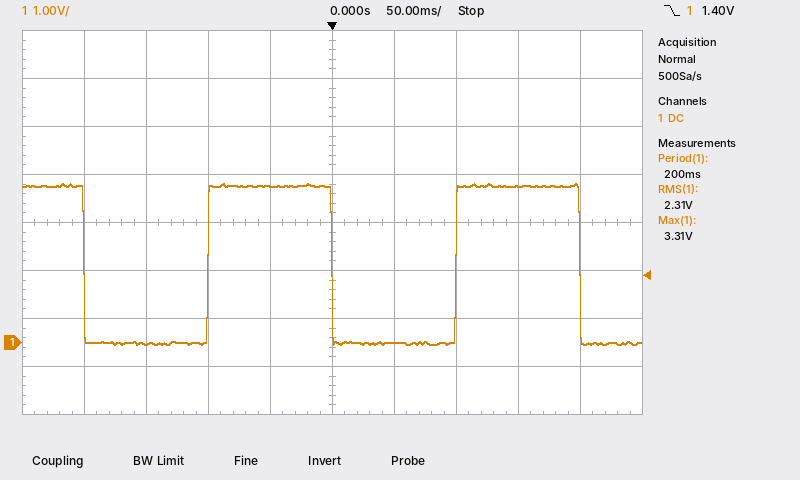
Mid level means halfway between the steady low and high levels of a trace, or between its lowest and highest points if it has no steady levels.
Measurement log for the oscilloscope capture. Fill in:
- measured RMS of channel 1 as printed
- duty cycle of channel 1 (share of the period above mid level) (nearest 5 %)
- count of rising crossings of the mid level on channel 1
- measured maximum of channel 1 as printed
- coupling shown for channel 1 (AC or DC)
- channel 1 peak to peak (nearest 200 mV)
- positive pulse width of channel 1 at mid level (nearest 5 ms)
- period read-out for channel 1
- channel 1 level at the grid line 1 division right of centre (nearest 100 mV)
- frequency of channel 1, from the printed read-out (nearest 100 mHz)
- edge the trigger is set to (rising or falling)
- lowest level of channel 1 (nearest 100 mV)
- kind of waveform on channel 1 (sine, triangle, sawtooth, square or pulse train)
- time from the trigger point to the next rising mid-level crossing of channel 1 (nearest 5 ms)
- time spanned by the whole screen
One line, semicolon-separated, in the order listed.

2.31 V; 50 %; 2; 3.31 V; DC; 3.4 V; 100 ms; 200 ms; 0.0 V; 5.0 Hz; falling; 0.0 V; square; 100 ms; 500 ms
